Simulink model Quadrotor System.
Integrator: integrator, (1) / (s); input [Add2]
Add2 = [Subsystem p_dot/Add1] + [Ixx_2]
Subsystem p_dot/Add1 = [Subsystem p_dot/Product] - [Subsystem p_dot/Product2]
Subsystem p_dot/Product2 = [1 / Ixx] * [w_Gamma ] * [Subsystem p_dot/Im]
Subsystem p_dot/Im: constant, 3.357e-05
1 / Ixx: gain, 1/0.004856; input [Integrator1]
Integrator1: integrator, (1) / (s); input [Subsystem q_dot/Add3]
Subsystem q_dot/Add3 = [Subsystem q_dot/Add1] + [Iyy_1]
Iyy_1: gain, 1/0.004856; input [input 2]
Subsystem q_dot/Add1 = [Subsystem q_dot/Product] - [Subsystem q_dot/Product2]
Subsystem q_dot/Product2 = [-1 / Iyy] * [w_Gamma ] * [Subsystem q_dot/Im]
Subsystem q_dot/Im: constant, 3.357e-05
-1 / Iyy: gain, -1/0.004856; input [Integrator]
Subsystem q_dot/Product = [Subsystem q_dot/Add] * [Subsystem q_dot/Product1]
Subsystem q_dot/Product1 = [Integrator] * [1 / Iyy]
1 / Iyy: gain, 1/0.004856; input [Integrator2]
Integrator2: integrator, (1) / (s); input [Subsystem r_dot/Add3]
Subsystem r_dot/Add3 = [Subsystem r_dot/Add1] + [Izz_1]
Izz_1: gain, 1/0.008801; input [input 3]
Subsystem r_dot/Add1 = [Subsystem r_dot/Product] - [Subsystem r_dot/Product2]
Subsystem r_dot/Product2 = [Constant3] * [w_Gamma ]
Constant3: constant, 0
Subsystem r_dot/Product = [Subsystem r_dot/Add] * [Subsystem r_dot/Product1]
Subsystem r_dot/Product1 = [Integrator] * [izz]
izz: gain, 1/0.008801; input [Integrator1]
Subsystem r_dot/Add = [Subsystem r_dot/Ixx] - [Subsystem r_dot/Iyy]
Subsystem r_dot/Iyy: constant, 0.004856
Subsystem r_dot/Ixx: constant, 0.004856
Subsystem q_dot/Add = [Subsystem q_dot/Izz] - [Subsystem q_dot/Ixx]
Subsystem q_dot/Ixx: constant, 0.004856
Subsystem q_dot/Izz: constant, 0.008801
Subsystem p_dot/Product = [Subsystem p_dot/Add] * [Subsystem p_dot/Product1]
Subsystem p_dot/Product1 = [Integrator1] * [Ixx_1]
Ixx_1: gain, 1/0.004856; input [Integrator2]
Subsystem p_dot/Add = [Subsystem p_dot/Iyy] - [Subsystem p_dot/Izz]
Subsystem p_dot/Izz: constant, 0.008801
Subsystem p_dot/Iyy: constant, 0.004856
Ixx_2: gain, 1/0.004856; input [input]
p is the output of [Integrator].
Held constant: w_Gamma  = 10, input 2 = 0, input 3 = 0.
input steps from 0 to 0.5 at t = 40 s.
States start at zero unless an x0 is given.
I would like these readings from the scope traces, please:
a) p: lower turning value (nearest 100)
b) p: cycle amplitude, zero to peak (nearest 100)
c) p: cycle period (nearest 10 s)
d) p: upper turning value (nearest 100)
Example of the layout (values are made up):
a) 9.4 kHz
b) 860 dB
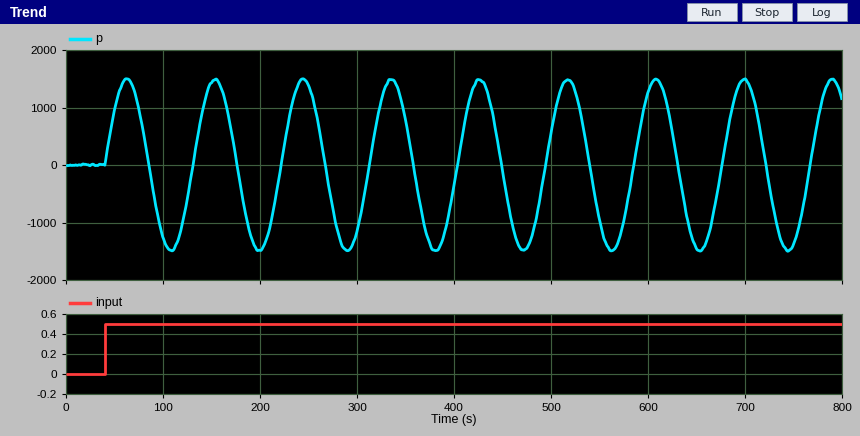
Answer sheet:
a) -1500
b) 1500
c) 90 s
d) 1500
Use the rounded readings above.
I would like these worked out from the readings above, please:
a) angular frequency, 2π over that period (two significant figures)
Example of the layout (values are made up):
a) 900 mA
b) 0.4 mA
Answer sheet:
a) 0.070 rad/s
